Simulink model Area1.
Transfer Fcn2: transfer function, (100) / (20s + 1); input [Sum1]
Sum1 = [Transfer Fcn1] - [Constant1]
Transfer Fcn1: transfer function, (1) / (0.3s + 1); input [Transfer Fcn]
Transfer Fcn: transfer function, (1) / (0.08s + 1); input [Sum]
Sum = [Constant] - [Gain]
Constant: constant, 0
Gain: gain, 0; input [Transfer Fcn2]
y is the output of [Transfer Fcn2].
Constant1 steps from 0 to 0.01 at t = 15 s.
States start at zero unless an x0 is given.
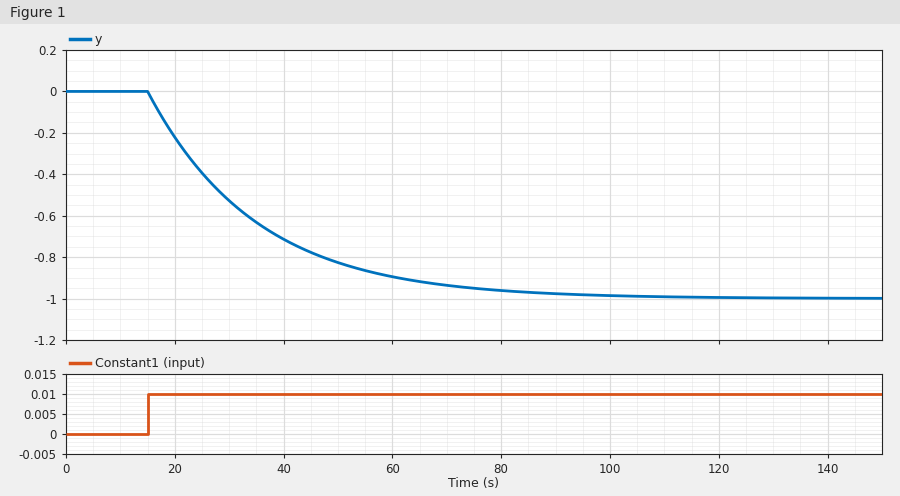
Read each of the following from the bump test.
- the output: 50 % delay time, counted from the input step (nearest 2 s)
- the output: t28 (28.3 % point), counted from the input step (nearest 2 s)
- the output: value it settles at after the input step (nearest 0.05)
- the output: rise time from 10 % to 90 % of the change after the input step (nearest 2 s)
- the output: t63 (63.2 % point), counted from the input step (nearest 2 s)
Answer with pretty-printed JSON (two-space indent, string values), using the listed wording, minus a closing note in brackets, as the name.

{
  "the output: 50 % delay time, counted from the input step": "14 s",
  "the output: t28 (28.3 % point), counted from the input step": "6 s",
  "the output: value it settles at after the input step": "-1.00",
  "the output: rise time from 10 % to 90 % of the change after the input step": "44 s",
  "the output: t63 (63.2 % point), counted from the input step": "20 s"
}
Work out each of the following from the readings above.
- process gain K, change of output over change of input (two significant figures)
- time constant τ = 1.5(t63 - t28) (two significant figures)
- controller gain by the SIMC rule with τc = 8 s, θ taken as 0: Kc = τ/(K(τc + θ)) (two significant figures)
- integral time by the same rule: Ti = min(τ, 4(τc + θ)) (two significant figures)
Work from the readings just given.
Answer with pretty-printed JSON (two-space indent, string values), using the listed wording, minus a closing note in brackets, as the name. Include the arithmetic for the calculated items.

{
  "process gain K, change of output over change of input": "(-1 - 0) / 0.01 = -100",
  "time constant τ = 1.5(t63 - t28)": "1.5 × (20 - 6) = 21 s",
  "controller gain by the SIMC rule with τc = 8 s, θ taken as 0: Kc = τ/(K(τc + θ))": "21 / (-100 × (8 + 0)) = -0.026",
  "integral time by the same rule: Ti = min(τ, 4(τc + θ))": "min(21, 4 × (8 + 0)) = 21 s"
}
